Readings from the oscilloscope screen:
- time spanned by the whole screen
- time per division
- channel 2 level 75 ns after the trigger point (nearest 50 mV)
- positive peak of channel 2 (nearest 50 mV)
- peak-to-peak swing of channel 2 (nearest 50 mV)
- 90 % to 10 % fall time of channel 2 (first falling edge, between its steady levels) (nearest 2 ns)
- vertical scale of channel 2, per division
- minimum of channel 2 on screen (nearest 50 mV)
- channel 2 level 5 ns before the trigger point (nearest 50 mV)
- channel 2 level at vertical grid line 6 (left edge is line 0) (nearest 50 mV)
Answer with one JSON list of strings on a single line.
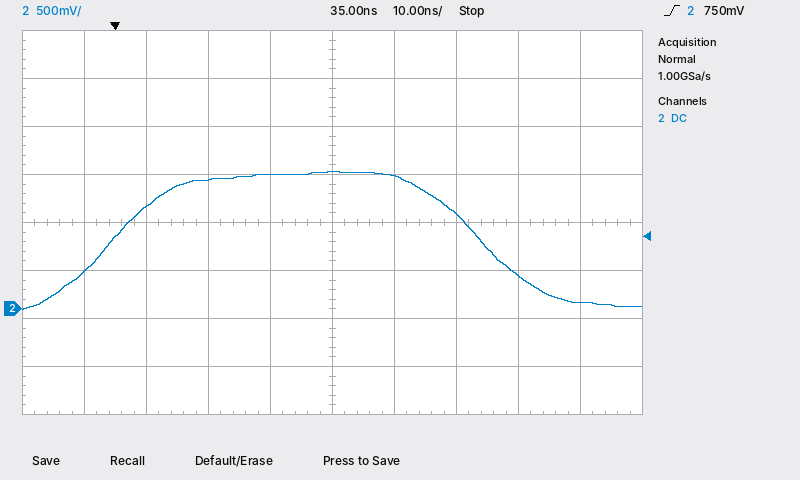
["100 ns", "10 ns", "50 mV", "1.45 V", "1.45 V", "20 ns", "500 mV", "0 mV", "400 mV", "1.40 V"]
